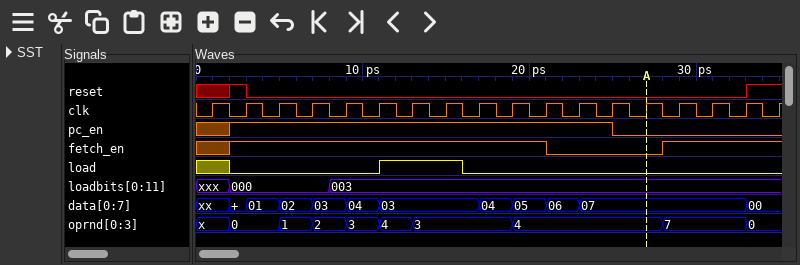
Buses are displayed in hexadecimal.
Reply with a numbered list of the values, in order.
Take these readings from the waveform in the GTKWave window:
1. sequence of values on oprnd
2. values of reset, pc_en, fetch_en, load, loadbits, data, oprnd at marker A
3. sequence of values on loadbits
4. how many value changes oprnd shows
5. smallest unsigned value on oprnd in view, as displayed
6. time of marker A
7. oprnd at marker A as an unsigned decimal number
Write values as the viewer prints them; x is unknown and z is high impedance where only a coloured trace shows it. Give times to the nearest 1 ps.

1. x, 0, 1, 2, 3, 4, 3, 4, 7, 0
2. reset=0, pc_en=0, fetch_en=0, load=0, loadbits=003, data=07, oprnd=4
3. xxx, 000, 003
4. 9
5. 0
6. 27 ps
7. 4
